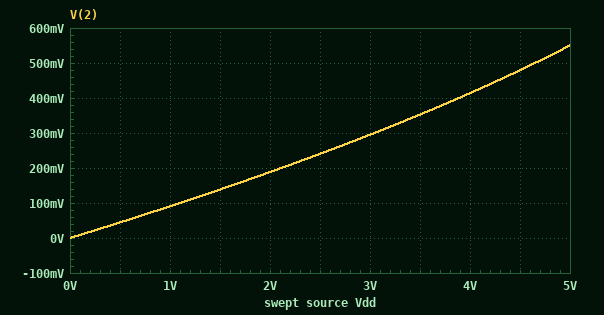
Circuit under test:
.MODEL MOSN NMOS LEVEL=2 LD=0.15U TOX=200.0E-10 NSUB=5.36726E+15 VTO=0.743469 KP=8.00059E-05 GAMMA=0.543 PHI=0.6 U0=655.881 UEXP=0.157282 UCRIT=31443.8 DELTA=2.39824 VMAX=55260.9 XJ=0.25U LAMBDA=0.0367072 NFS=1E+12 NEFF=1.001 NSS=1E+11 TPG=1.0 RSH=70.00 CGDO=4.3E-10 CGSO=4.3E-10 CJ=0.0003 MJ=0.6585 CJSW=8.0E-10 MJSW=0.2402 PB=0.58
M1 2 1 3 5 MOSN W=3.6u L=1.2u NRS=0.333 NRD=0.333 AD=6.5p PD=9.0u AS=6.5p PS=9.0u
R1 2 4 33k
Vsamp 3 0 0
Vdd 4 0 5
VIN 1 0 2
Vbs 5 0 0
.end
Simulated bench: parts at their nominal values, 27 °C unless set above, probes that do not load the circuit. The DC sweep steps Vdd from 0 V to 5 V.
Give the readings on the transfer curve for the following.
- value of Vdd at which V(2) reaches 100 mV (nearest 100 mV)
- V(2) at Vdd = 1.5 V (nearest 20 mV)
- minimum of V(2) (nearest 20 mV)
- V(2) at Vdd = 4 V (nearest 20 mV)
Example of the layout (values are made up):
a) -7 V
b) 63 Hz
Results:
a) 1.1 V
b) 140 mV
c) 0 V
d) 420 mV
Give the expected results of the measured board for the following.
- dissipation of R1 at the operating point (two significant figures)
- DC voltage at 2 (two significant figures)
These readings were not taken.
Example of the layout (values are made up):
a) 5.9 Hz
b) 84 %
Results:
a) 600 µW
b) 550 mV
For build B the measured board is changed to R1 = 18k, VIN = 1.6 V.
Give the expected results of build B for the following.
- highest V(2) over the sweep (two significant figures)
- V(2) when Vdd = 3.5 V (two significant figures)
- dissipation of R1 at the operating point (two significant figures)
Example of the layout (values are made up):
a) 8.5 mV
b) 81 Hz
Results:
a) 3.2 V
b) 1.8 V
c) 190 µW
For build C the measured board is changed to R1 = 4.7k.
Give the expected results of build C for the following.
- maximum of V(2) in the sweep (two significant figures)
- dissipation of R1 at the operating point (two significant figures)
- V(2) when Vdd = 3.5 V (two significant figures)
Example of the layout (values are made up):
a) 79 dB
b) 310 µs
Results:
a) 4.1 V
b) 160 µW
c) 2.7 V
